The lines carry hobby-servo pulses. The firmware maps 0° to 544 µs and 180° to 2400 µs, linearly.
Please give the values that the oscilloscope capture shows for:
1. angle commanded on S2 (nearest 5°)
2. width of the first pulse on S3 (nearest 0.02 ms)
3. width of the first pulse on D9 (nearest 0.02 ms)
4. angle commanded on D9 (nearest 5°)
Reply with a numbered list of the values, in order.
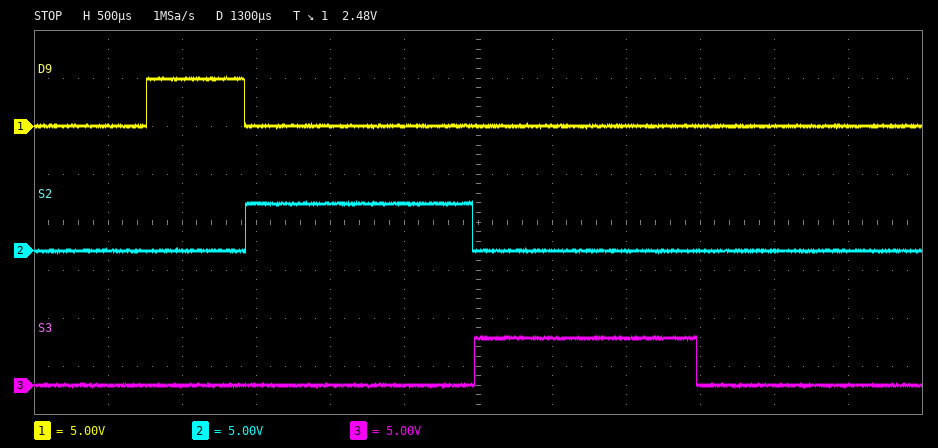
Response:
1. 95°
2. 1.50 ms
3. 0.66 ms
4. 10°
